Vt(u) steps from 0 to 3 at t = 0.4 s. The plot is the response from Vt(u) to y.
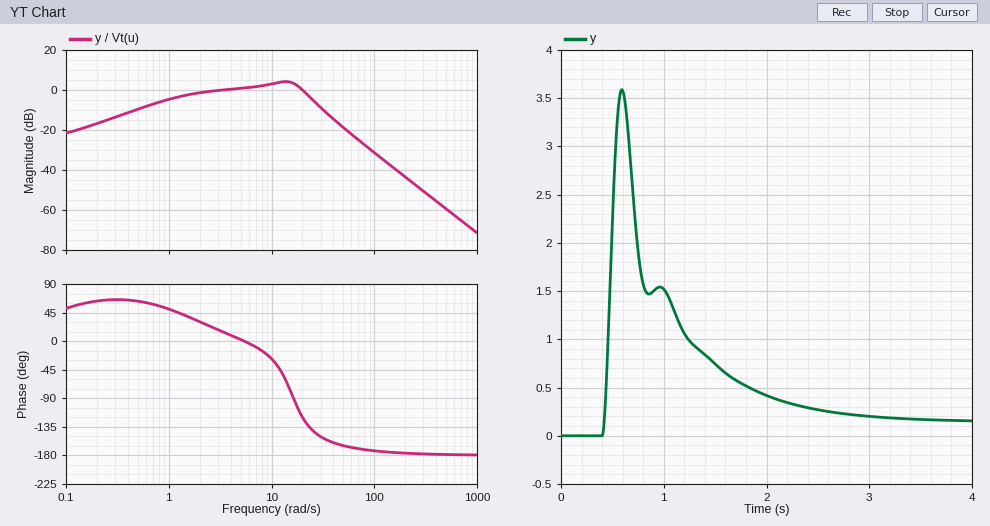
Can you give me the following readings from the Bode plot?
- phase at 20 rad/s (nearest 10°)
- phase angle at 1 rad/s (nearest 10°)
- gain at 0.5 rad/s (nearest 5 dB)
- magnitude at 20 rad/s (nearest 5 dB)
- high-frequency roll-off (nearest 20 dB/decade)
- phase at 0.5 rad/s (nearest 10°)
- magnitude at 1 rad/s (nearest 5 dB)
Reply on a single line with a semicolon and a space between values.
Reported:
-120°; 50°; -10 dB; 0 dB; -40 dB/decade; 60°; -5 dB
